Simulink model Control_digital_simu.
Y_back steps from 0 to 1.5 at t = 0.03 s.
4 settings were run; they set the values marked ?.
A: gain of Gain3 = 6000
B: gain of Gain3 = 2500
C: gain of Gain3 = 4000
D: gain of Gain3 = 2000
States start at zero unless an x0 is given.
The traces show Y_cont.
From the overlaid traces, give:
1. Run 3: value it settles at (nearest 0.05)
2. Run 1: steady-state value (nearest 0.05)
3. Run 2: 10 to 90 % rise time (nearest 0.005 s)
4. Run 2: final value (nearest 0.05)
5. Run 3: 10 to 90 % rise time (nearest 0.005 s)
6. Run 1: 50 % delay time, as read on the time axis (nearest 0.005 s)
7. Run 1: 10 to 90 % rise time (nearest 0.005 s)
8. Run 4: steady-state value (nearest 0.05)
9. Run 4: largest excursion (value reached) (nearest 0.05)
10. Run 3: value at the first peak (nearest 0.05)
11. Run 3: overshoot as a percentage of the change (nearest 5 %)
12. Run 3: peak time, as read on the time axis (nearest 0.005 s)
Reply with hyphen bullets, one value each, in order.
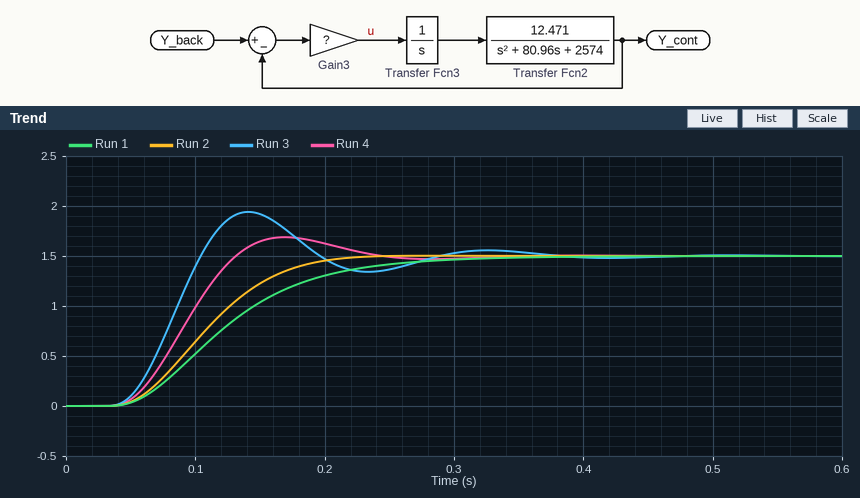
- 1.50
- 1.50
- 0.105 s
- 1.50
- 0.045 s
- 0.120 s
- 0.150 s
- 1.50
- 1.70
- 1.95
- 30 %
- 0.140 s
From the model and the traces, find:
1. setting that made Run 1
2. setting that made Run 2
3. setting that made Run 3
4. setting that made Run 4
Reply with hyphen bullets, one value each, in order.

- D
- B
- A
- C
